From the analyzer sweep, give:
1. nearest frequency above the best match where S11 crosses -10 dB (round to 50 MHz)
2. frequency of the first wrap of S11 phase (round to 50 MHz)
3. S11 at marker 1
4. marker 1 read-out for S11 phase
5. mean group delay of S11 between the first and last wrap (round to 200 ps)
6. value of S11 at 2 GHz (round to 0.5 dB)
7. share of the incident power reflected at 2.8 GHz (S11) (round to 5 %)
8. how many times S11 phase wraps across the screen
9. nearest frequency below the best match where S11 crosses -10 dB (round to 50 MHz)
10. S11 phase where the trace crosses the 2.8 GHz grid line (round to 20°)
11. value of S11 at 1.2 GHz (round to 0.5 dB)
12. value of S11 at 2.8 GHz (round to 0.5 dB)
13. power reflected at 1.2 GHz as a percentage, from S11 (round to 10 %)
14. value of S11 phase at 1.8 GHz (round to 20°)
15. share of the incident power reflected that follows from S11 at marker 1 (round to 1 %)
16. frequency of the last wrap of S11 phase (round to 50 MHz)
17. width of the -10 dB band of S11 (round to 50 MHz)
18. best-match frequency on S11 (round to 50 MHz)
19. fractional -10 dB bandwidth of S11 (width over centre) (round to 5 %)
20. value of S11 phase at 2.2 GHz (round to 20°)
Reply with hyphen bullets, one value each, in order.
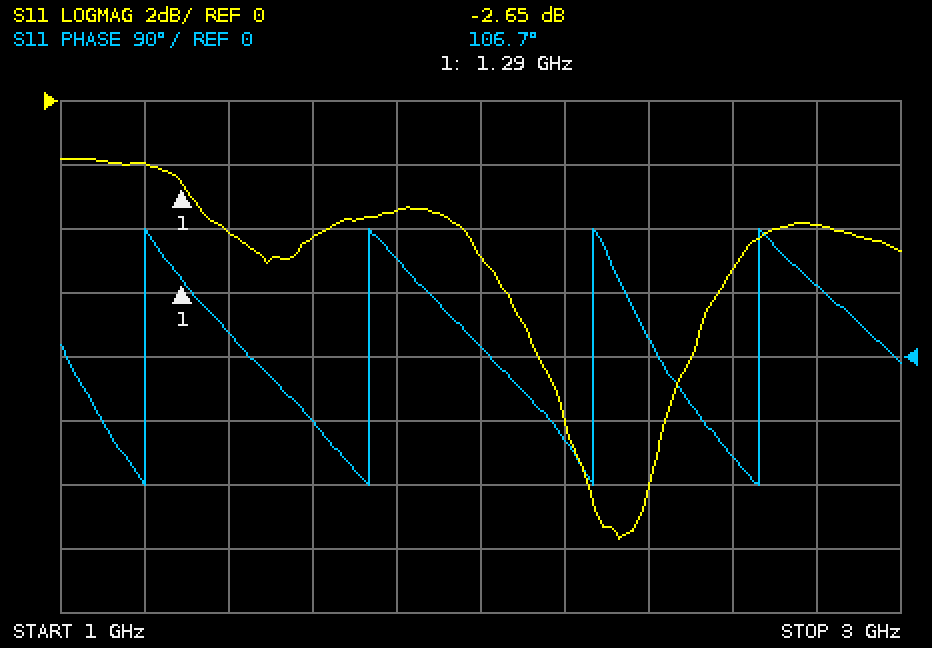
- 2.45 GHz
- 1.20 GHz
- -2.65 dB
- 106.7°
- 2.0 ns
- -5.0 dB
- 40 %
- 4
- 2.20 GHz
- 100°
- -2.0 dB
- -4.0 dB
- 60 %
- 140°
- 54 %
- 2.65 GHz
- 250 MHz
- 2.35 GHz
- 10 %
- -120°
